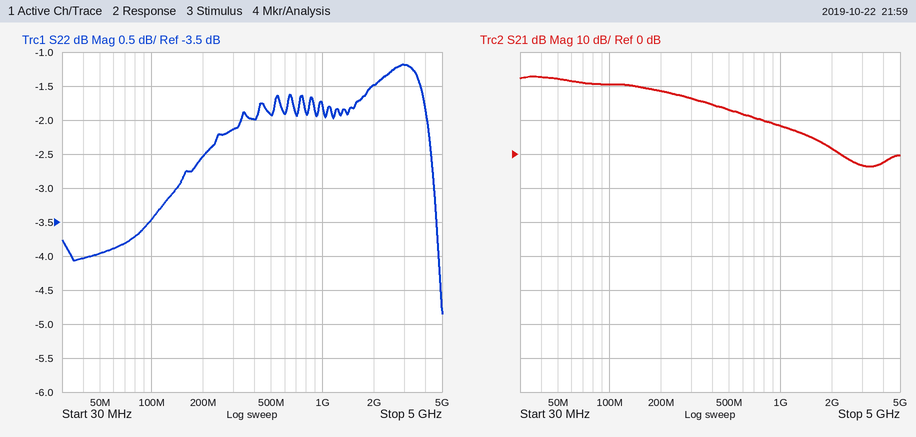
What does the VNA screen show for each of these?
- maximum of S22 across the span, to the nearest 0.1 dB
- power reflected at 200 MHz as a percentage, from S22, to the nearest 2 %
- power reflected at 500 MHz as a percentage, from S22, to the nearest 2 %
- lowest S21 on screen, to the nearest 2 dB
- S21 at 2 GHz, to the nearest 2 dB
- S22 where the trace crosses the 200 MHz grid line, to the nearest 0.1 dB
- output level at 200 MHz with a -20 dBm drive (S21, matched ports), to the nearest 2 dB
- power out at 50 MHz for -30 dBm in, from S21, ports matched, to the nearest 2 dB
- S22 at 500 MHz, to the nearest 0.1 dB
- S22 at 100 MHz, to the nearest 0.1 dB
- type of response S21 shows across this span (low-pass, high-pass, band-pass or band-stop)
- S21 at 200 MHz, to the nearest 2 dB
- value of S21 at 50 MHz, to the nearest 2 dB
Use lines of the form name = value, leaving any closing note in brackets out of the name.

maximum of S22 across the span, to the nearest 0.1 dB = -1.2 dB
power reflected at 200 MHz as a percentage, from S22, to the nearest 2 % = 56 %
power reflected at 500 MHz as a percentage, from S22, to the nearest 2 % = 64 %
lowest S21 on screen, to the nearest 2 dB = -4 dB
S21 at 2 GHz, to the nearest 2 dB = 2 dB
S22 where the trace crosses the 200 MHz grid line, to the nearest 0.1 dB = -2.5 dB
output level at 200 MHz with a -20 dBm drive (S21, matched ports), to the nearest 2 dB = -2 dBm
power out at 50 MHz for -30 dBm in, from S21, ports matched, to the nearest 2 dB = -8 dBm
S22 at 500 MHz, to the nearest 0.1 dB = -1.9 dB
S22 at 100 MHz, to the nearest 0.1 dB = -3.5 dB
type of response S21 shows across this span = low-pass
S21 at 200 MHz, to the nearest 2 dB = 18 dB
value of S21 at 50 MHz, to the nearest 2 dB = 22 dB
